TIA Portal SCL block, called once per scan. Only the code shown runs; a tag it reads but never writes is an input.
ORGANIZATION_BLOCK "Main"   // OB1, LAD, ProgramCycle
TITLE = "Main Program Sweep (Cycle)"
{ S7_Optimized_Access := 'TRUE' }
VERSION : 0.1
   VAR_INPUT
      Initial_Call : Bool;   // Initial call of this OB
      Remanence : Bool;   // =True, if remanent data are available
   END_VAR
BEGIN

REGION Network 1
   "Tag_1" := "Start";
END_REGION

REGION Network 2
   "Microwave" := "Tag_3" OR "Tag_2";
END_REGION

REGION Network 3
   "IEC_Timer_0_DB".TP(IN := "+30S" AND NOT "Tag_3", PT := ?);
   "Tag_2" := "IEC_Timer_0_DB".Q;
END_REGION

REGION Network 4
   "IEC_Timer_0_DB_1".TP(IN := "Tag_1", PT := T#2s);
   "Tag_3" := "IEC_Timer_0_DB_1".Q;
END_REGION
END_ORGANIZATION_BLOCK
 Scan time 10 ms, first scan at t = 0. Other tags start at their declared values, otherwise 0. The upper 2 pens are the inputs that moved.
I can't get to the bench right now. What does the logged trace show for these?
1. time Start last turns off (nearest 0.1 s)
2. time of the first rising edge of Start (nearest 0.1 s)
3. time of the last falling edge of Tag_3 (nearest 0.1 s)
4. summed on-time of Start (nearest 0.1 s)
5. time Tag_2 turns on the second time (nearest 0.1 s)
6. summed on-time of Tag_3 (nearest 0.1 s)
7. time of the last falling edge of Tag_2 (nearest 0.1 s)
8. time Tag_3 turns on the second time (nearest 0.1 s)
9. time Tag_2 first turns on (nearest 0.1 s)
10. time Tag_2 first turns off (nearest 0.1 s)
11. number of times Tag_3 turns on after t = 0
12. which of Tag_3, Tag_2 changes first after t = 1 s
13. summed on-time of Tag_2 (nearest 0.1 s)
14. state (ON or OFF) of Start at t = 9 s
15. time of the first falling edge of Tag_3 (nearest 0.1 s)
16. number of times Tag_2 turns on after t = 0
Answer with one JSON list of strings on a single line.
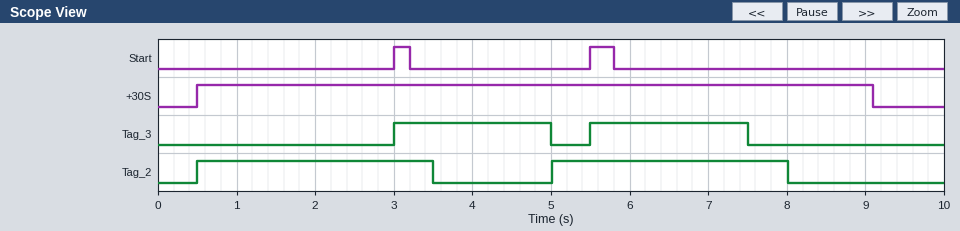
["5.8 s", "3.0 s", "7.5 s", "0.5 s", "5.0 s", "4.0 s", "8.0 s", "5.5 s", "0.5 s", "3.5 s", "2", "Tag_3", "6.0 s", "OFF", "5.0 s", "2"]
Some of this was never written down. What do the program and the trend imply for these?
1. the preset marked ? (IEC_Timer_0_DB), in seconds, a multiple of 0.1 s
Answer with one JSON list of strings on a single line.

["3.0 s"]
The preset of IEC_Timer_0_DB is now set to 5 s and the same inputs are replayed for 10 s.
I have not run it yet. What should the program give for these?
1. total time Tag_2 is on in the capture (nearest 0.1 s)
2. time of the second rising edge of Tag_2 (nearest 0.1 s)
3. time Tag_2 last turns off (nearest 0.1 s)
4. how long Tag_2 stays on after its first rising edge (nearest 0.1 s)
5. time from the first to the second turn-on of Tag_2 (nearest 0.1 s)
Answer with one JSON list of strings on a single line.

["7.5 s", "7.5 s", "5.5 s", "5.0 s", "7.0 s"]
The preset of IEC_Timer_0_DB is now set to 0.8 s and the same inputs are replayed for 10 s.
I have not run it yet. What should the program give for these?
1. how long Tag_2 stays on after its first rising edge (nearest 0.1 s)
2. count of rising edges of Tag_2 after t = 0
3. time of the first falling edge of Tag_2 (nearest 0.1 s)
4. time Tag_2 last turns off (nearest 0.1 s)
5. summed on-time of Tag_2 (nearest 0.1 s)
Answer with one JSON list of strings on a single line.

["0.8 s", "3", "1.3 s", "8.3 s", "2.4 s"]
